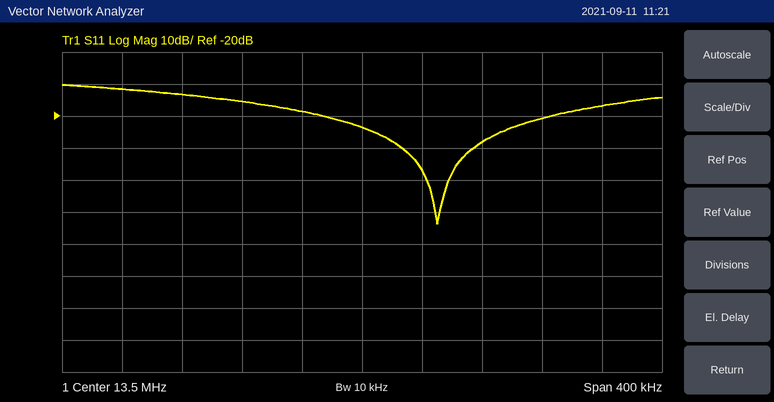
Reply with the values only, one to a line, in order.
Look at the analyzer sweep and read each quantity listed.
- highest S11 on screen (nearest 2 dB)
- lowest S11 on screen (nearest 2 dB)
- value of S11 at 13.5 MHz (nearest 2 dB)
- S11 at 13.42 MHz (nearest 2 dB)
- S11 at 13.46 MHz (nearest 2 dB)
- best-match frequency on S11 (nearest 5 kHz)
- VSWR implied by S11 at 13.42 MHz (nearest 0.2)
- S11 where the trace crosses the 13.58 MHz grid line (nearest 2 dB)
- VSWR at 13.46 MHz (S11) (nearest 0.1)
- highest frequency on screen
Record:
-10 dB
-54 dB
-24 dB
-16 dB
-18 dB
13.550 MHz
1.4
-28 dB
1.3
13.7 MHz
